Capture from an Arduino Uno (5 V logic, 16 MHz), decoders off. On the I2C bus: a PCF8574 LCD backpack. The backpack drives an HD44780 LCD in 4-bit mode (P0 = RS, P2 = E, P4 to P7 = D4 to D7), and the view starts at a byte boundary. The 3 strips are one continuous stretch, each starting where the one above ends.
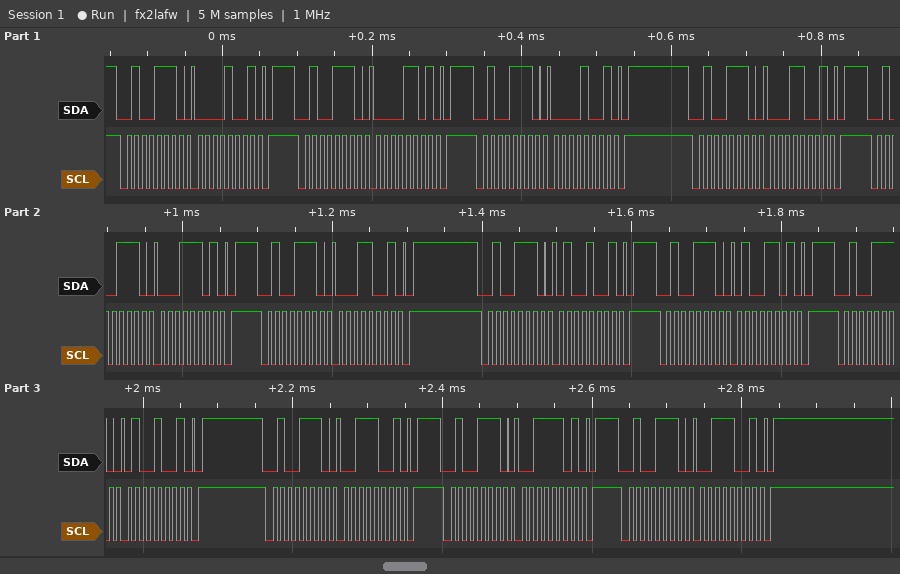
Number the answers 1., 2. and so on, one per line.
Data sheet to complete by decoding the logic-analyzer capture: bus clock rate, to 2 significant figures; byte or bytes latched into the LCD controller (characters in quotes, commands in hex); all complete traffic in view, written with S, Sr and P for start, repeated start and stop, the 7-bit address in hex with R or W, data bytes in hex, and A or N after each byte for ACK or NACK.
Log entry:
1. 100 kHz
2. data 0x01 'C'
3. S 27W A 09 A P S 27W A 0D A P S 27W A 09 A P S 27W A 19 A P S 27W A 1D A P S 27W A 19 A P S 27W A 49 A P S 27W A 4D A P S 27W A 49 A P S 27W A 39 A P S 27W A 3D A P S 27W A 39 A P
